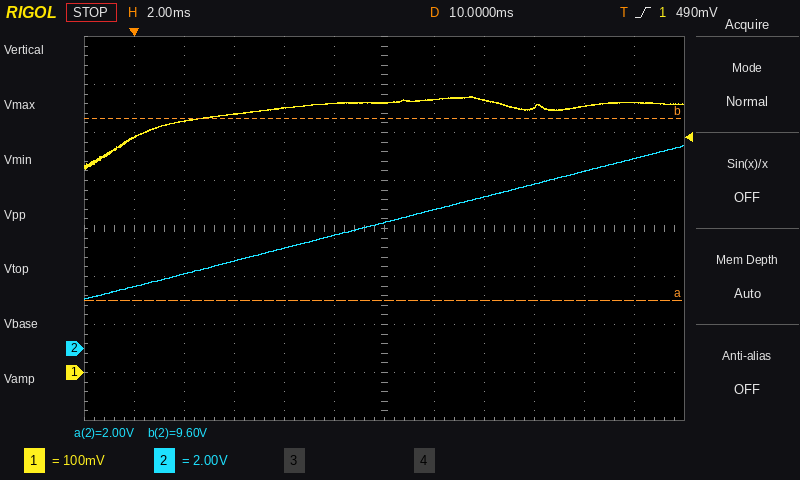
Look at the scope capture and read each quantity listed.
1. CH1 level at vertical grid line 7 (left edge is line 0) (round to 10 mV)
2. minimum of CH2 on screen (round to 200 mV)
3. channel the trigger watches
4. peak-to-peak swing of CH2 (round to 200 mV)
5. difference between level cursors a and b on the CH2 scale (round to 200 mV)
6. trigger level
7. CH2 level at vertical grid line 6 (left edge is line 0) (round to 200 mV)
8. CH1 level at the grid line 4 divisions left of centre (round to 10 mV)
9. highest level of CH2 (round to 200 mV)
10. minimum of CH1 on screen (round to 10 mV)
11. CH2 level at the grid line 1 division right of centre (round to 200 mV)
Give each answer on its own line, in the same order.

570 mV
2.0 V
CH1
6.4 V
7.6 V
490 mV
5.2 V
520 mV
8.4 V
420 mV
5.8 V
